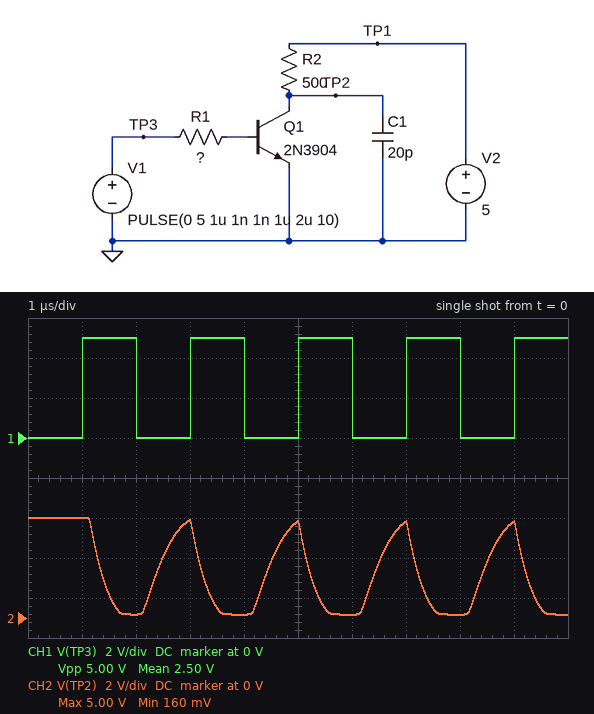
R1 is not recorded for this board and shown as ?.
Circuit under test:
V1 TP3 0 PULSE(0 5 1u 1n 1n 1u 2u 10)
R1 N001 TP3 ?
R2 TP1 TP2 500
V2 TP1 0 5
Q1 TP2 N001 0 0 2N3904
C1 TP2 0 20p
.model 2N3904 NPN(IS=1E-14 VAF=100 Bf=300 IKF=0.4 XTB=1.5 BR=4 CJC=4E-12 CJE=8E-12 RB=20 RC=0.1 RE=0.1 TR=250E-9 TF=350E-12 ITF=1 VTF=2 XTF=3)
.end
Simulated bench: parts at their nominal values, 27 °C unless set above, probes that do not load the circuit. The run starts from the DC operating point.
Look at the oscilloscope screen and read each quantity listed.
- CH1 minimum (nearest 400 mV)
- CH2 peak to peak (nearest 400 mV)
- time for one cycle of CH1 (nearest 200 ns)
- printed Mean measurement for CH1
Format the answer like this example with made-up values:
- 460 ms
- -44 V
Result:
- 0 V
- 4.8 V
- 2.0 µs
- 2.50 V
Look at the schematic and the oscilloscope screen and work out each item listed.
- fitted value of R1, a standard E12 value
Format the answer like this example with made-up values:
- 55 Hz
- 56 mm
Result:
- 82 kΩ
